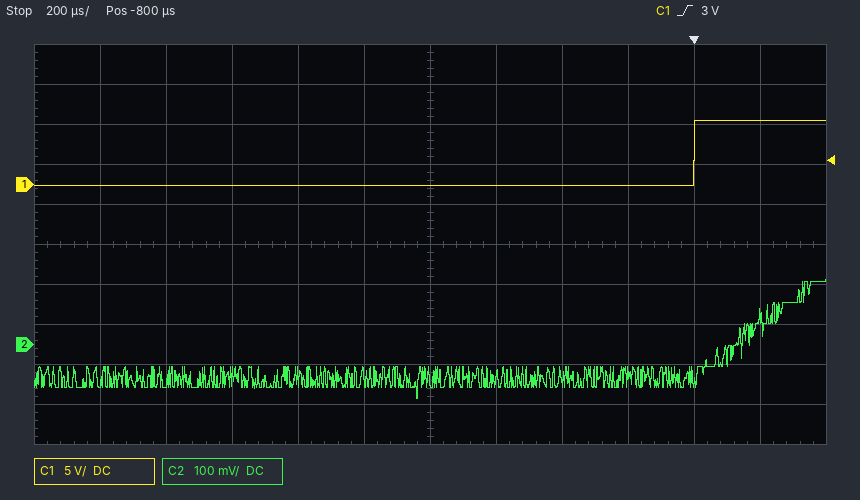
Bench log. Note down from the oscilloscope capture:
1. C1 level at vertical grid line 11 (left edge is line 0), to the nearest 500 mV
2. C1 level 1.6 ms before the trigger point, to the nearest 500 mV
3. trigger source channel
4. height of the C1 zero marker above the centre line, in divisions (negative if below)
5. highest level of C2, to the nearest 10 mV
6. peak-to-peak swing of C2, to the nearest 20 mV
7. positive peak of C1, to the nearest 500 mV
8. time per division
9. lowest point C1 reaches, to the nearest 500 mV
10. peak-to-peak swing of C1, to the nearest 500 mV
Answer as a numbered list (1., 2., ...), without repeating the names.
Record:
1. 8.0 V
2. 0.0 V
3. C1
4. +1.5 div
5. 160 mV
6. 300 mV
7. 8.0 V
8. 200 µs
9. 0.0 V
10. 8.0 V
